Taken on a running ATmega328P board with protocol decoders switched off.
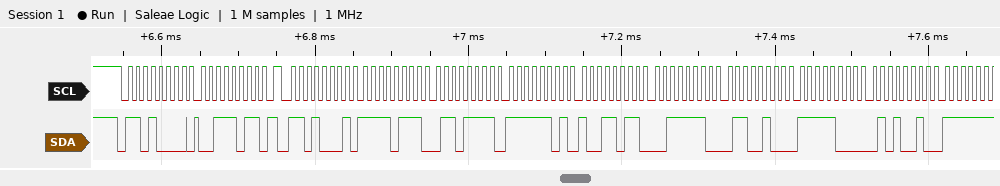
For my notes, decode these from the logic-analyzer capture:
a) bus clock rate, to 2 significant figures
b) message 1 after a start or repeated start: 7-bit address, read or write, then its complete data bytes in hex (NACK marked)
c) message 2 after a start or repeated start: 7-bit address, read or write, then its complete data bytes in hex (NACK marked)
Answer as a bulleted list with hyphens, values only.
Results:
- 100 kHz
- 0x68 write: 3B
- 0x68 read: F7 6F FD 9B 3E 64 F8 52
